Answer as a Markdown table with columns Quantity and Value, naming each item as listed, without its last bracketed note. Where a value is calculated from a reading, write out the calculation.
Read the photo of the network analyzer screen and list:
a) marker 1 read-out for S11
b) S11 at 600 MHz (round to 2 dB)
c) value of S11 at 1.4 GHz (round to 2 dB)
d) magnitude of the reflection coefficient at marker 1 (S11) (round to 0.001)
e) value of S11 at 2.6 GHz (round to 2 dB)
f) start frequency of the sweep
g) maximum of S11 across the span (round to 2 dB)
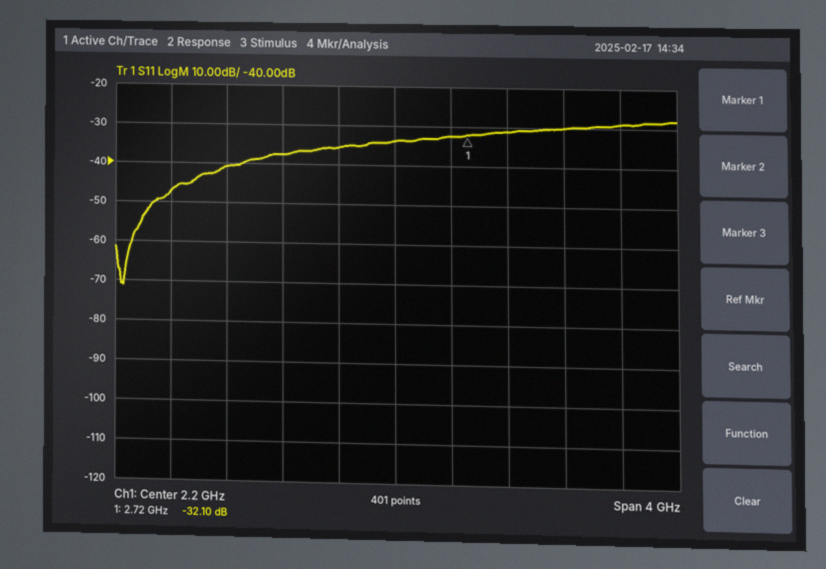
| Quantity | Value |
|---|---|
| marker 1 read-out for S11 | -32.10 dB |
| S11 at 600 MHz | -48 dB |
| value of S11 at 1.4 GHz | -38 dB |
| magnitude of the reflection coefficient at marker 1 (S11) | 10^(-32.1/20) ≈ 0.025 |
| value of S11 at 2.6 GHz | -32 dB |
| start frequency of the sweep | 200 MHz |
| maximum of S11 across the span | -28 dB |
